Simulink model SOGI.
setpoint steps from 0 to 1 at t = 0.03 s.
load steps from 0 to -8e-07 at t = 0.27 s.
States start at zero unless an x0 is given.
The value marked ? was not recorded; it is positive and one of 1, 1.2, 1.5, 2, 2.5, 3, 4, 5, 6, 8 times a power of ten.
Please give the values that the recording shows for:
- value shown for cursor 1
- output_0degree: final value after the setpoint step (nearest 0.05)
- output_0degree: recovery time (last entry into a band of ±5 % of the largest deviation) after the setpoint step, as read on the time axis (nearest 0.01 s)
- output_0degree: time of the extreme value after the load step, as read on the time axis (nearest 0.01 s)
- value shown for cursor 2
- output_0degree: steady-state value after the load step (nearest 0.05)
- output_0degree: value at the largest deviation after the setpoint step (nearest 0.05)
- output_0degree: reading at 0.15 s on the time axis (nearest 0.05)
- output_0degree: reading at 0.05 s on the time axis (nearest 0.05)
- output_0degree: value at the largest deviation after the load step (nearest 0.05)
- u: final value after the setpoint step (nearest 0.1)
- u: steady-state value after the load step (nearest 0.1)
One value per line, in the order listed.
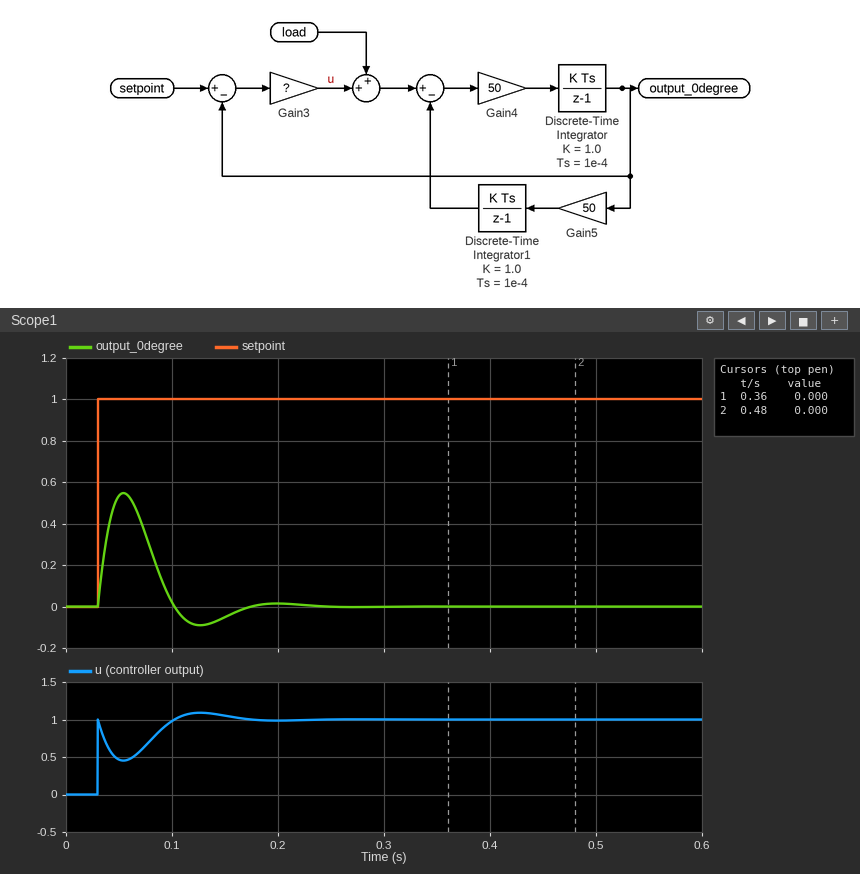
0.000
0.00
0.16 s
0.34 s
0.000
0.00
0.55
-0.05
0.55
0.00
1.0
1.0
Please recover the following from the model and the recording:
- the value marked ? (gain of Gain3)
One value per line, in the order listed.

1
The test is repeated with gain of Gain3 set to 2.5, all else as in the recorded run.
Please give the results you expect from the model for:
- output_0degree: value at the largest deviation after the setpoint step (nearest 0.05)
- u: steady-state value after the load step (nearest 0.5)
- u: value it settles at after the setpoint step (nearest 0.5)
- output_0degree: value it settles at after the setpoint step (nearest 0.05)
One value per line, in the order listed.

0.80
2.5
2.5
0.00
